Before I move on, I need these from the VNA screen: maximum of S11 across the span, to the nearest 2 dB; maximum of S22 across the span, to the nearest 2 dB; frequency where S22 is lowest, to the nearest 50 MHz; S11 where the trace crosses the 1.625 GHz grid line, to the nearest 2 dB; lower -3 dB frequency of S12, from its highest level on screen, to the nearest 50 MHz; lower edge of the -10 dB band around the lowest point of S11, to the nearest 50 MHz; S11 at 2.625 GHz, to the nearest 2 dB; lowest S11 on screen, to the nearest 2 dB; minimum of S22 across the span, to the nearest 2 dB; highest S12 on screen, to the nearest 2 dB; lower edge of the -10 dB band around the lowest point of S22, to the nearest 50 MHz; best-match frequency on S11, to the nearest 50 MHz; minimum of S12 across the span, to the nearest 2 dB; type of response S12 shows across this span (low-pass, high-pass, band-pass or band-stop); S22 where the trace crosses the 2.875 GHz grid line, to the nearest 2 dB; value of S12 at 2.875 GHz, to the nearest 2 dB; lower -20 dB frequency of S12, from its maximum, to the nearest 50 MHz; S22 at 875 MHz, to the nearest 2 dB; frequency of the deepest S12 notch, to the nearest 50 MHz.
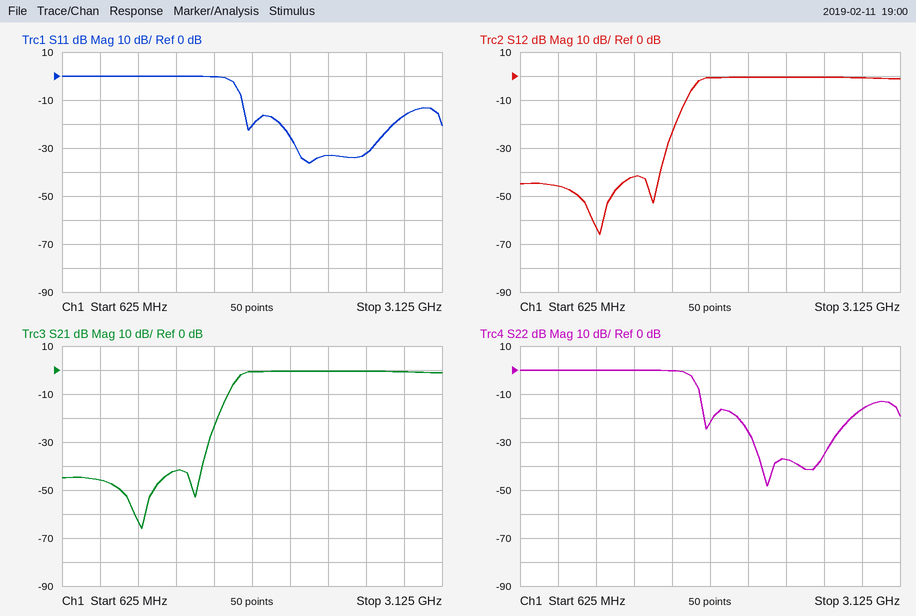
0 dB
0 dB
2.25 GHz
0 dB
1.80 GHz
1.80 GHz
-32 dB
-36 dB
-48 dB
0 dB
1.80 GHz
2.25 GHz
-66 dB
high-pass
-16 dB
0 dB
1.65 GHz
0 dB
1.15 GHz
